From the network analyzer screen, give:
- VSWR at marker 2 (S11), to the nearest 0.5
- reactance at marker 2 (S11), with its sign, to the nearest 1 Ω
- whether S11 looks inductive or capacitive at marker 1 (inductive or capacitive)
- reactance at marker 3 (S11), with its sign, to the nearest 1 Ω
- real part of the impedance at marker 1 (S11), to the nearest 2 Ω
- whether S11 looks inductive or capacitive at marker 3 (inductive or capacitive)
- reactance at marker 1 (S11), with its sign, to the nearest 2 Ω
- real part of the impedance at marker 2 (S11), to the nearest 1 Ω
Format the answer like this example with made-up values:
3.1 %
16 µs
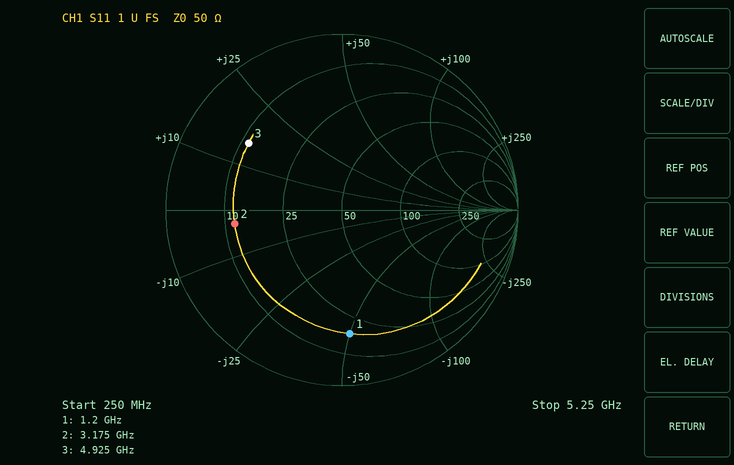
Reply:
4.0
-3 Ω
capacitive
+15 Ω
18 Ω
inductive
-50 Ω
12 Ω
